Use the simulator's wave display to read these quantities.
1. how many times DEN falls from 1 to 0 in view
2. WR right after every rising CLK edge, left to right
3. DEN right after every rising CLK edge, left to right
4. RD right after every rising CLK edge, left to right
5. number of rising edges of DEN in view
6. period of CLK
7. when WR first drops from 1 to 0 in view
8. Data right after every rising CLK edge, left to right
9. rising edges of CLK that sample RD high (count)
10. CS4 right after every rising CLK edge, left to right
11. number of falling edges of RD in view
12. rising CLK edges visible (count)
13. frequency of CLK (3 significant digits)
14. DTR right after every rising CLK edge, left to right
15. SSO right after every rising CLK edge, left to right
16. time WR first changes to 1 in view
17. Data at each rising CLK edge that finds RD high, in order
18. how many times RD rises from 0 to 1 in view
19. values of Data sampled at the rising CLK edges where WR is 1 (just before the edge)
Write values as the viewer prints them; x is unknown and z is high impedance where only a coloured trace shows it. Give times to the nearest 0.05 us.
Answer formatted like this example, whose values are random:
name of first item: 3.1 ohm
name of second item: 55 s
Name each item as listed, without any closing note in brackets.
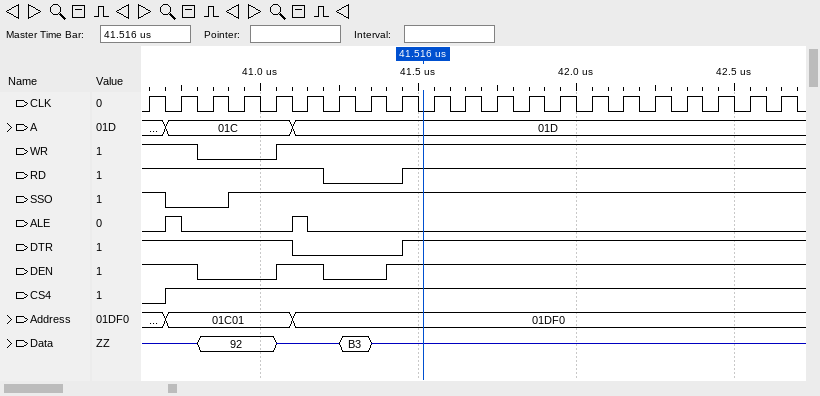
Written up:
how many times DEN falls from 1 to 0 in view: 2
WR right after every rising CLK edge, left to right: 1 1 0 0 1 1 1 1 1 1 1 1 1 1 1 1 1 1 1 1 1
DEN right after every rising CLK edge, left to right: 1 1 0 0 1 1 0 0 1 1 1 1 1 1 1 1 1 1 1 1 1
RD right after every rising CLK edge, left to right: 1 1 1 1 1 1 0 0 1 1 1 1 1 1 1 1 1 1 1 1 1
number of rising edges of DEN in view: 2
period of CLK: 0.1 us
when WR first drops from 1 to 0 in view: 40.8 us
Data right after every rising CLK edge, left to right: z, z, 92, 92, z, z, B3, z, z, z, z, z, z, z, z, z, z, z, z, z, z
rising edges of CLK that sample RD high: 18
CS4 right after every rising CLK edge, left to right: 0 1 1 1 1 1 1 1 1 1 1 1 1 1 1 1 1 1 1 1 1
number of falling edges of RD in view: 1
rising CLK edges visible: 21
frequency of CLK: 10.0 MHz
DTR right after every rising CLK edge, left to right: 1 1 1 1 1 0 0 0 1 1 1 1 1 1 1 1 1 1 1 1 1
SSO right after every rising CLK edge, left to right: 1 0 0 1 1 1 1 1 1 1 1 1 1 1 1 1 1 1 1 1 1
time WR first changes to 1 in view: 41.05 us
Data at each rising CLK edge that finds RD high, in order: z, z, 92, 92, 92, z, z, z, z, z, z, z, z, z, z, z, z, z
how many times RD rises from 0 to 1 in view: 1
values of Data sampled at the rising CLK edges where WR is 1: z, z, z, z, B3, z, z, z, z, z, z, z, z, z, z, z, z, z
